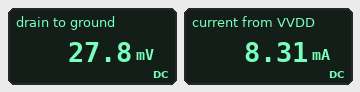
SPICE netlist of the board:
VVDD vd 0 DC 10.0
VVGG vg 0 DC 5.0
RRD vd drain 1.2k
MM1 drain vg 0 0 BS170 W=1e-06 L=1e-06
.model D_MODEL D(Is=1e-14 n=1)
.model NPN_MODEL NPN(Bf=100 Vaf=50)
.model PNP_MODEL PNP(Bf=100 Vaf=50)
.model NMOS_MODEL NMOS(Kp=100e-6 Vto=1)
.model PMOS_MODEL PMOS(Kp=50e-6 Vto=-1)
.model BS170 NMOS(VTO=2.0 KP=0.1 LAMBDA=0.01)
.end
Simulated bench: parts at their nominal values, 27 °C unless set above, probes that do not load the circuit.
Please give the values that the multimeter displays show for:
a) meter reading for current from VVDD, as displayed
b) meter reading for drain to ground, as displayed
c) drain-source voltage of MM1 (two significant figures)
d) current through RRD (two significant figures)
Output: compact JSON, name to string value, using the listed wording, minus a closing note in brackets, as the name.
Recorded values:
{"meter reading for current from VVDD, as displayed": "8.31 mA", "meter reading for drain to ground, as displayed": "27.8 mV", "drain-source voltage of MM1": "28 mV", "current through RRD": "8.3 mA"}
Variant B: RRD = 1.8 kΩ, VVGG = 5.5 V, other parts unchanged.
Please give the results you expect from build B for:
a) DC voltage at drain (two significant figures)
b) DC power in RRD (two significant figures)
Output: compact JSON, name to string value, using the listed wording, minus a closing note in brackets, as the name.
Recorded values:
{"DC voltage at drain": "16 mV", "DC power in RRD": "55 mW"}
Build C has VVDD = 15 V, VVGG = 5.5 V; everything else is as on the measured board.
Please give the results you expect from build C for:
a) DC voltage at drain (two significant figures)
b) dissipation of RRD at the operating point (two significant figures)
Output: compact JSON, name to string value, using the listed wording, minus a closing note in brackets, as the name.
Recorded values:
{"DC voltage at drain": "36 mV", "dissipation of RRD at the operating point": "190 mW"}
